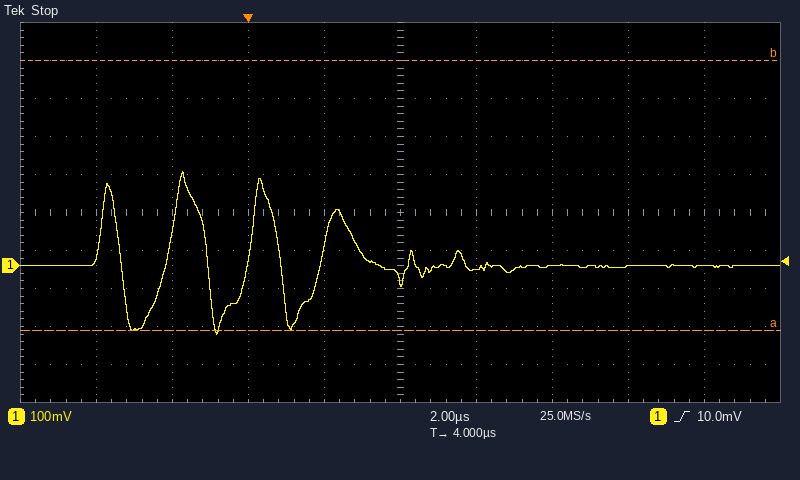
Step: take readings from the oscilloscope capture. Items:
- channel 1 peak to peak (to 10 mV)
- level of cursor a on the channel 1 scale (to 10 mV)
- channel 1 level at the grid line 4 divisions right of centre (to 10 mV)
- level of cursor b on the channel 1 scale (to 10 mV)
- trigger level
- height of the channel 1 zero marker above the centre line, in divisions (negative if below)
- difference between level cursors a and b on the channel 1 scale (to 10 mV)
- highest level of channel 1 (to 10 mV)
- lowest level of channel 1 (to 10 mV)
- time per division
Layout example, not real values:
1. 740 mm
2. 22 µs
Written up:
1. 430 mV
2. -170 mV
3. 0 mV
4. 540 mV
5. 10.0 mV
6. -1.4 div
7. 710 mV
8. 250 mV
9. -180 mV
10. 2 µs
